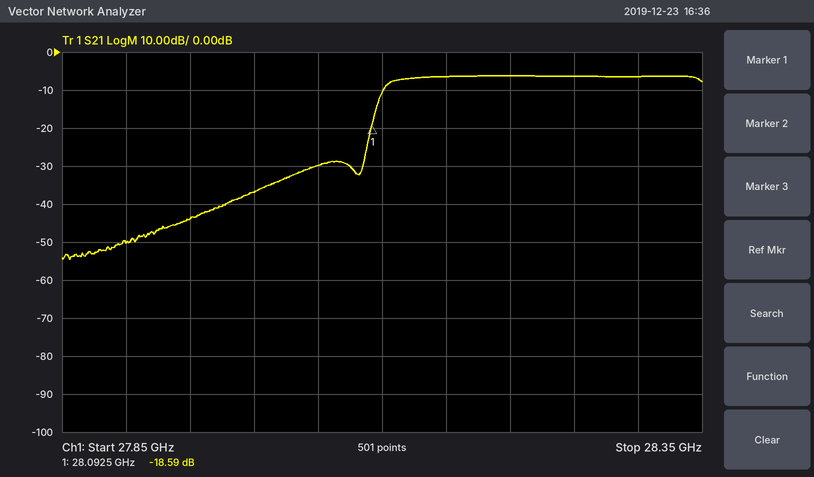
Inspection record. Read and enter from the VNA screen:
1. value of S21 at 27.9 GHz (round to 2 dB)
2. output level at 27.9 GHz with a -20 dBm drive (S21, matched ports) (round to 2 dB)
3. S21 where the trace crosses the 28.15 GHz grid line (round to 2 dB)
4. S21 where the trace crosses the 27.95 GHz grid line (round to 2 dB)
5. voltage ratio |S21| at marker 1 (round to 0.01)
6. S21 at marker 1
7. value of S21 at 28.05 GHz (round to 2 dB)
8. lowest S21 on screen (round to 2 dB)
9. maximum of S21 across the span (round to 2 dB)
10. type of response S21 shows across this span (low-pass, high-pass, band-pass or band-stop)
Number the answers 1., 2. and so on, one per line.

1. -50 dB
2. -70 dBm
3. -6 dB
4. -44 dB
5. 0.12
6. -18.59 dB
7. -30 dB
8. -54 dB
9. -6 dB
10. high-pass
